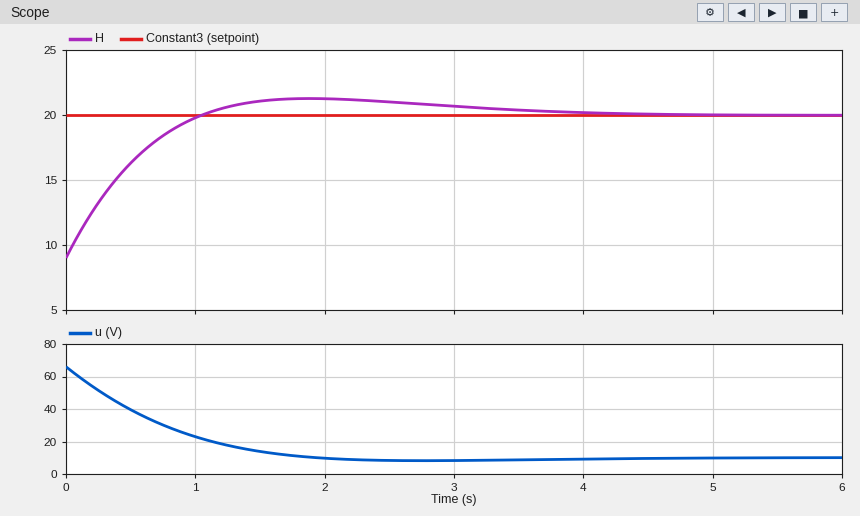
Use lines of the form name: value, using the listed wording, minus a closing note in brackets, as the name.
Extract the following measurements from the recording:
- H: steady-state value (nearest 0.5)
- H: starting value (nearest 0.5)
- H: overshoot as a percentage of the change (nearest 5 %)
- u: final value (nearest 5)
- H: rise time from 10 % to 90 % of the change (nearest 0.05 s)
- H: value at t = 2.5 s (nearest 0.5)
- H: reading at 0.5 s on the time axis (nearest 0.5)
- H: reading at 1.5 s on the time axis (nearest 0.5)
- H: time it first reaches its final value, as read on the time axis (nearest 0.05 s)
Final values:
H: steady-state value: 20.0
H: starting value: 9.0
H: overshoot as a percentage of the change: 10 %
u: final value: 10
H: rise time from 10 % to 90 % of the change: 0.75 s
H: value at t = 2.5 s: 21.0
H: reading at 0.5 s on the time axis: 16.5
H: reading at 1.5 s on the time axis: 21.0
H: time it first reaches its final value, as read on the time axis: 1.05 s
